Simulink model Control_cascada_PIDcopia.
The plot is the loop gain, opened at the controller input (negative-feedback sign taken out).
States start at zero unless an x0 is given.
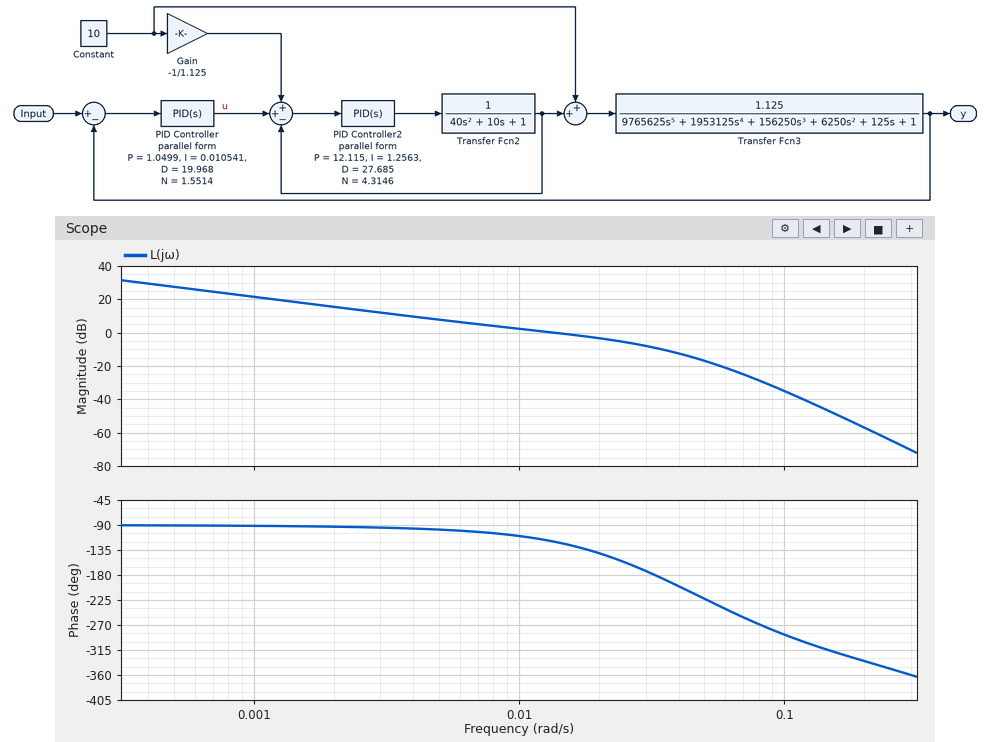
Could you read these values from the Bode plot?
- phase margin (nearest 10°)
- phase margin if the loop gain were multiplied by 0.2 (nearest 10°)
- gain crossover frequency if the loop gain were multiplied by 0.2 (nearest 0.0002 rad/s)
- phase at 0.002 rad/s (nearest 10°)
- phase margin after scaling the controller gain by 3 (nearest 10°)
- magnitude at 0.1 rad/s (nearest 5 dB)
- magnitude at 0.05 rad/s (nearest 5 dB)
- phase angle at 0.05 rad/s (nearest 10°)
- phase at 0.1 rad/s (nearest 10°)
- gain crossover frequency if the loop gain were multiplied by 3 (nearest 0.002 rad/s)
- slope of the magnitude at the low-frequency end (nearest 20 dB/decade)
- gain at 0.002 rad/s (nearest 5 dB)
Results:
60°
90°
0.0024 rad/s
-90°
0°
-35 dB
-15 dB
-220°
-290°
0.034 rad/s
-20 dB/decade
15 dB
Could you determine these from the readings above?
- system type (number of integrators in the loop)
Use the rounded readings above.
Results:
1
